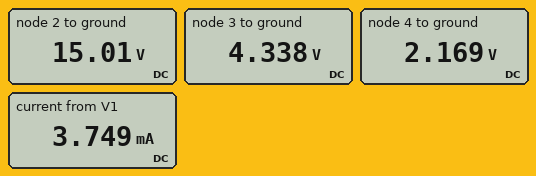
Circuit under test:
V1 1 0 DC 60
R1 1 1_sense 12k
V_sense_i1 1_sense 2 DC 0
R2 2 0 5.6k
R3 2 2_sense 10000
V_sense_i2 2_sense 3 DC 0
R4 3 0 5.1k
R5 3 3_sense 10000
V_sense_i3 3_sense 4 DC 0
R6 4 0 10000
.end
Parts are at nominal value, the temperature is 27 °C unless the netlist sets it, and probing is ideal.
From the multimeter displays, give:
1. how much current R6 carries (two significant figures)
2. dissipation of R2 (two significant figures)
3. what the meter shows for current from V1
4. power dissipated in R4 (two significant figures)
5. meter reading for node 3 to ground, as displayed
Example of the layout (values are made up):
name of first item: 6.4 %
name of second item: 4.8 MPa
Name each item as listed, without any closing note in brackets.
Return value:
how much current R6 carries: 220 µA
dissipation of R2: 40 mW
what the meter shows for current from V1: 3.749 mA
power dissipated in R4: 3.7 mW
meter reading for node 3 to ground, as displayed: 4.338 V
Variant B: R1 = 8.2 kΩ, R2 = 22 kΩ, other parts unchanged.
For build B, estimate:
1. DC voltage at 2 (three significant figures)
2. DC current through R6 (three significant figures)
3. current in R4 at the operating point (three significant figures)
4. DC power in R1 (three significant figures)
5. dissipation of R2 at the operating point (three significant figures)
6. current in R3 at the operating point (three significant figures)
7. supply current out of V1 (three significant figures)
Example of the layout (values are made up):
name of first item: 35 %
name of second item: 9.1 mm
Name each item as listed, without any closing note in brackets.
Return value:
DC voltage at 2: 30.7 V
DC current through R6: 443 µA
current in R4 at the operating point: 1.74 mA
DC power in R1: 105 mW
dissipation of R2 at the operating point: 42.8 mW
current in R3 at the operating point: 2.18 mA
supply current out of V1: 3.58 mA
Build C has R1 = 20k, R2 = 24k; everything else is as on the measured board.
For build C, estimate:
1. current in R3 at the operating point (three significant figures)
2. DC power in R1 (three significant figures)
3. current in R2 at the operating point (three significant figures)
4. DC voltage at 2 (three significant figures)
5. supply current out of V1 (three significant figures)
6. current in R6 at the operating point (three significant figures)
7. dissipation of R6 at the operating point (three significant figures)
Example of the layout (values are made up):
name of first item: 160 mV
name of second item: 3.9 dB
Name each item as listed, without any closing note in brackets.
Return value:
current in R3 at the operating point: 1.31 mA
DC power in R1: 86.4 mW
current in R2 at the operating point: 768 µA
DC voltage at 2: 18.4 V
supply current out of V1: 2.08 mA
current in R6 at the operating point: 266 µA
dissipation of R6 at the operating point: 709 µW
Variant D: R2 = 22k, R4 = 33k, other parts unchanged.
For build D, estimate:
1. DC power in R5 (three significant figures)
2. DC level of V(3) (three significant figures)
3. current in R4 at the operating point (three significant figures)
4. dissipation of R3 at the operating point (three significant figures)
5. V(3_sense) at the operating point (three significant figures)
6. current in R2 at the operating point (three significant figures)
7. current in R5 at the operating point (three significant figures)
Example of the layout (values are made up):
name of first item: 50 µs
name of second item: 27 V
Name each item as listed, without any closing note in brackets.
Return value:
DC power in R5: 6.40 mW
DC level of V(3): 16.0 V
current in R4 at the operating point: 485 µA
dissipation of R3 at the operating point: 16.5 mW
V(3_sense) at the operating point: 8.00 V
current in R2 at the operating point: 1.31 mA
current in R5 at the operating point: 800 µA
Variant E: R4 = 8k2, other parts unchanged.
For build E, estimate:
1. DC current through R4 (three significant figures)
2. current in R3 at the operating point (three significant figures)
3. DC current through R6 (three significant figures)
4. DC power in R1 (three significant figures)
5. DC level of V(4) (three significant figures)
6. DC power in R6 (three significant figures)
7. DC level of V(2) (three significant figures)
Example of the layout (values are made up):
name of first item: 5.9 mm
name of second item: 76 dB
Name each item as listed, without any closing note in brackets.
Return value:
DC current through R4: 690 µA
current in R3 at the operating point: 972 µA
DC current through R6: 283 µA
DC power in R1: 166 mW
DC level of V(4): 2.83 V
DC power in R6: 799 µW
DC level of V(2): 15.4 V
